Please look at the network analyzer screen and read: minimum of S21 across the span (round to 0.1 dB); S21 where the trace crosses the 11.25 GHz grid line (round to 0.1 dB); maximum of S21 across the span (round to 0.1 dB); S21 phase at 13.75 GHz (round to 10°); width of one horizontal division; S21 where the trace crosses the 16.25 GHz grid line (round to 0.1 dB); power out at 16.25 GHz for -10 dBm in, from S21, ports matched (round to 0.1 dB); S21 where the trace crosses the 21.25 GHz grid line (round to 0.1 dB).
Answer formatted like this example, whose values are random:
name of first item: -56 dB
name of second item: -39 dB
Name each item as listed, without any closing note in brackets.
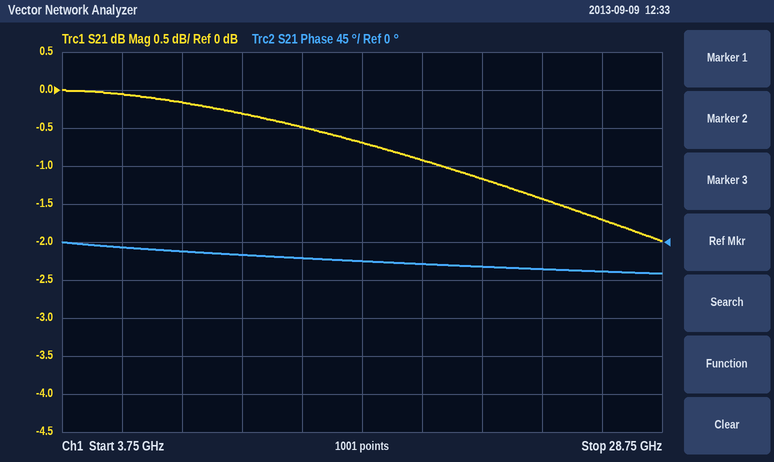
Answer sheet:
minimum of S21 across the span: -2.0 dB
S21 where the trace crosses the 11.25 GHz grid line: -0.3 dB
maximum of S21 across the span: 0.0 dB
S21 phase at 13.75 GHz: -20°
width of one horizontal division: 2.5 GHz
S21 where the trace crosses the 16.25 GHz grid line: -0.7 dB
power out at 16.25 GHz for -10 dBm in, from S21, ports matched: -10.7 dBm
S21 where the trace crosses the 21.25 GHz grid line: -1.2 dB
